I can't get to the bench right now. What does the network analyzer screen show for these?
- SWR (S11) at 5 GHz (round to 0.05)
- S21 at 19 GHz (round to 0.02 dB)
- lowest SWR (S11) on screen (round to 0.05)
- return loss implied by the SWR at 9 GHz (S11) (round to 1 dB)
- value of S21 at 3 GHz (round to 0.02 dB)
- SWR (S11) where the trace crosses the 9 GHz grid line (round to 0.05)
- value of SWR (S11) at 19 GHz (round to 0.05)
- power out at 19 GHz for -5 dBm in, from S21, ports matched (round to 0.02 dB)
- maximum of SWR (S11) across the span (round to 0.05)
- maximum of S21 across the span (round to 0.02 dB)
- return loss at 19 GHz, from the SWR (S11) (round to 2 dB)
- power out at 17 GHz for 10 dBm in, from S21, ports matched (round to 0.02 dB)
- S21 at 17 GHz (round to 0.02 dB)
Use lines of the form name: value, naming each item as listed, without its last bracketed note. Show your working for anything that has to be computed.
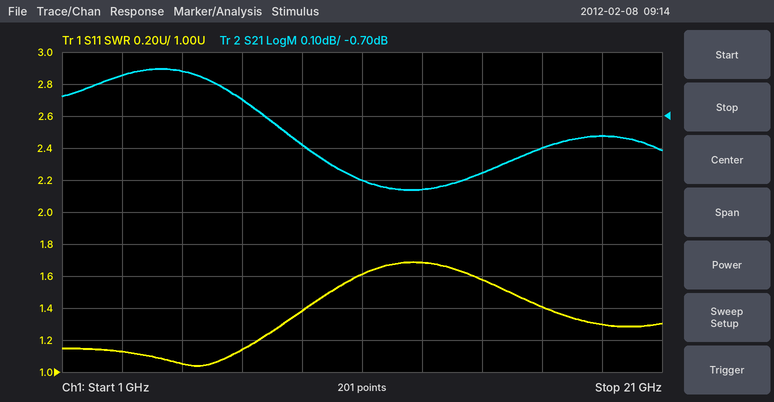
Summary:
SWR (S11) at 5 GHz: 1.05
S21 at 19 GHz: -0.76 dB
lowest SWR (S11) on screen: 1.05
return loss implied by the SWR at 9 GHz (S11): −20 log10((1.4 − 1)/(1.4 + 1)) ≈ 16 dB
value of S21 at 3 GHz: -0.58 dB
SWR (S11) where the trace crosses the 9 GHz grid line: 1.40
value of SWR (S11) at 19 GHz: 1.30
power out at 19 GHz for -5 dBm in, from S21, ports matched: -5 dBm + (-0.76 dB) = -5.76 dBm
maximum of SWR (S11) across the span: 1.70
maximum of S21 across the span: -0.56 dB
return loss at 19 GHz, from the SWR (S11): −20 log10((1.3 − 1)/(1.3 + 1)) ≈ 18 dB
power out at 17 GHz for 10 dBm in, from S21, ports matched: 10 dBm + (-0.80 dB) = 9.20 dBm
S21 at 17 GHz: -0.80 dB
